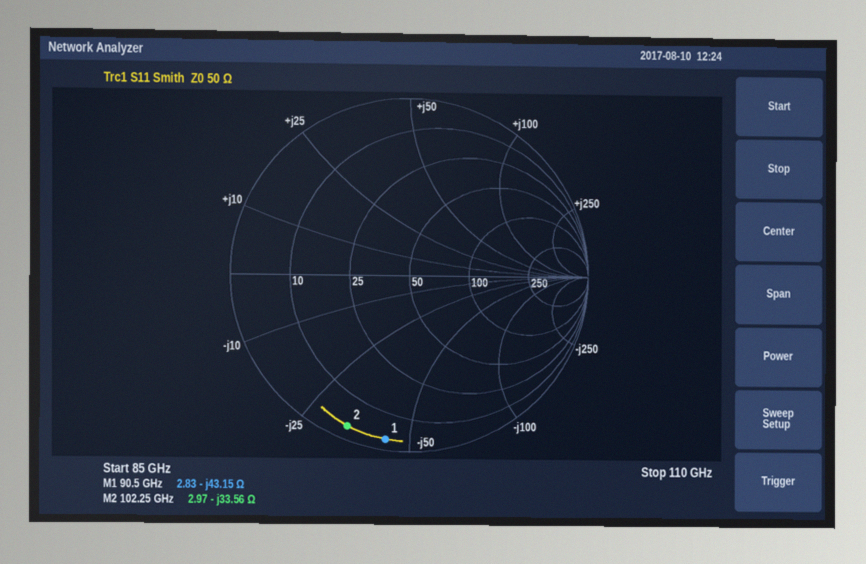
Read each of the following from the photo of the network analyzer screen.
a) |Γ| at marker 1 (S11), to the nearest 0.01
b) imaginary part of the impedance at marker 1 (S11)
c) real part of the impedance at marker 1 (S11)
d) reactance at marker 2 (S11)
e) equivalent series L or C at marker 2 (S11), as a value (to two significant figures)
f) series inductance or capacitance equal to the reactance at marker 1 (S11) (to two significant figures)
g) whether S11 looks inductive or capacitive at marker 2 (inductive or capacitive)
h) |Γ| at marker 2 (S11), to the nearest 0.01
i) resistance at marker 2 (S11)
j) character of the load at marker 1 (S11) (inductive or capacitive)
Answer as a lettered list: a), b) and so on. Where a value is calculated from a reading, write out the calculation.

a) 0.94
b) -43.15 Ω
c) 2.83 Ω
d) -33.56 Ω
e) C = 1/(2π × 102.25 GHz × 33.56 Ω) ≈ 46 fF
f) C = 1/(2π × 90.5 GHz × 43.15 Ω) ≈ 41 fF
g) capacitive
h) 0.92
i) 2.97 Ω
j) capacitive
